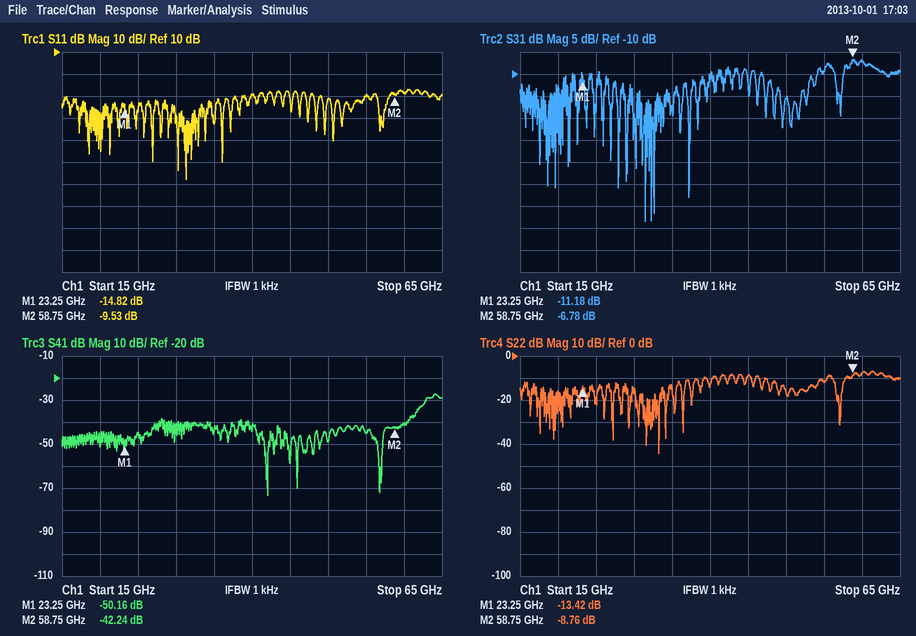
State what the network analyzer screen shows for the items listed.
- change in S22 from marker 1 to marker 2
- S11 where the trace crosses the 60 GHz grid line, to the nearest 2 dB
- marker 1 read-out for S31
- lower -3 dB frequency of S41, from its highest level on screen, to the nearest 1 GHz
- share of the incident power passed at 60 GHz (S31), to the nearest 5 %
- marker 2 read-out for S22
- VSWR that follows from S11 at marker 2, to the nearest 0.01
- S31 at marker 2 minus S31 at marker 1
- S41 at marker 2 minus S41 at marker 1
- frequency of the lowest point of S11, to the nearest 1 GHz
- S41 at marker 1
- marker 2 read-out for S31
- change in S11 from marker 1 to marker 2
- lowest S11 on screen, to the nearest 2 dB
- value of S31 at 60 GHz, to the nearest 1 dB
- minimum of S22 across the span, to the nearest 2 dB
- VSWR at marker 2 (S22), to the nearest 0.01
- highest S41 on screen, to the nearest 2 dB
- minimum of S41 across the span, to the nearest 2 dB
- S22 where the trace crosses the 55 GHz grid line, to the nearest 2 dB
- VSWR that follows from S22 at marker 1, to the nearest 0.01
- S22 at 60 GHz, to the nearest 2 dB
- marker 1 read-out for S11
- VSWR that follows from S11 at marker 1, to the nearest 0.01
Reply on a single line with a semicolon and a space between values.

4.66 dB; -8 dB; -11.18 dB; 63 GHz; 20 %; -8.76 dB; 2.00; 4.40 dB; 7.92 dB; 31 GHz; -50.16 dB; -6.78 dB; 5.29 dB; -48 dB; -7 dB; -44 dB; 2.15; -28 dB; -74 dB; -12 dB; 1.54; -8 dB; -14.82 dB; 1.44
